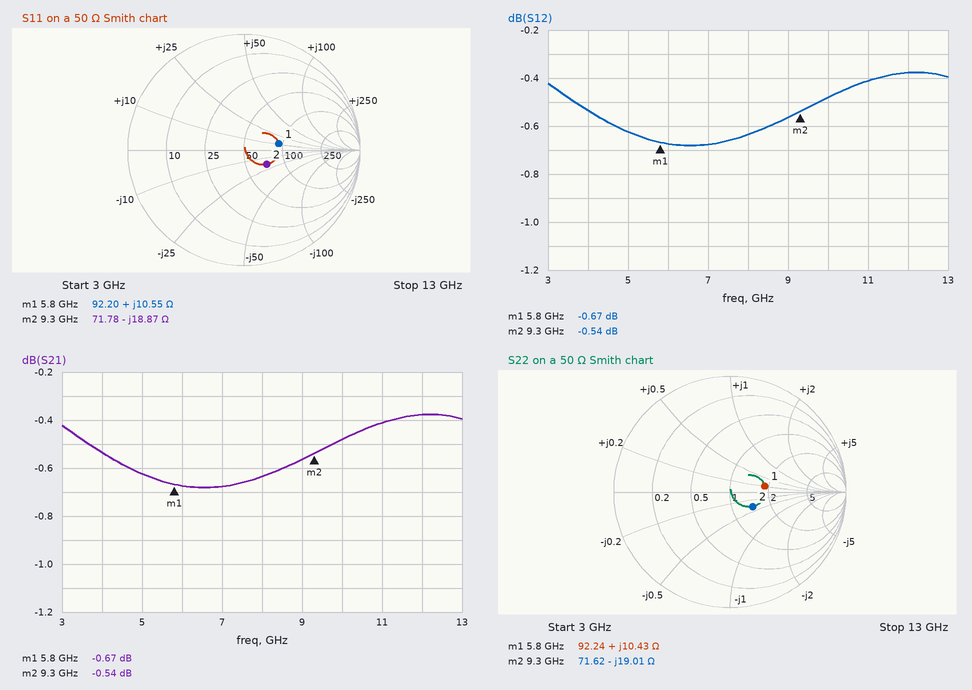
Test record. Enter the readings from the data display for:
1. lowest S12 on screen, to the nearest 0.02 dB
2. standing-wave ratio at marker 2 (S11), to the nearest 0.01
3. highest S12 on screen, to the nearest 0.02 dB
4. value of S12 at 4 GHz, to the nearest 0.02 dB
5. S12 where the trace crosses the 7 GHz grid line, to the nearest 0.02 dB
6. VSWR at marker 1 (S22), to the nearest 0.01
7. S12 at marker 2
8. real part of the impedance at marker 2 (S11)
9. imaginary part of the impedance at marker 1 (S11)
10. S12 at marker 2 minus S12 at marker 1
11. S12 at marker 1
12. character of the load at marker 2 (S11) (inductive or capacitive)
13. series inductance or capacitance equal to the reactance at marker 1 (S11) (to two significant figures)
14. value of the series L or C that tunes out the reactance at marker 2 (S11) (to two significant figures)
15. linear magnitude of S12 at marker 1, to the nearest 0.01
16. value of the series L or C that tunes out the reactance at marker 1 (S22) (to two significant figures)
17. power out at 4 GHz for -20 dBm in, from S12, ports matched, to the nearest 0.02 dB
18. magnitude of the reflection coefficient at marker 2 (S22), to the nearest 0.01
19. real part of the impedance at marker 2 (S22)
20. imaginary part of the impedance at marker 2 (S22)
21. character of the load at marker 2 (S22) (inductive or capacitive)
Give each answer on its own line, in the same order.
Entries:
-0.68 dB
1.61
-0.38 dB
-0.54 dB
-0.68 dB
1.88
-0.54 dB
71.78 Ω
+10.55 Ω
0.13 dB
-0.67 dB
capacitive
290 pH
320 pH
0.93
2.6 pF
-20.54 dBm
0.23
71.62 Ω
-19.01 Ω
capacitive
